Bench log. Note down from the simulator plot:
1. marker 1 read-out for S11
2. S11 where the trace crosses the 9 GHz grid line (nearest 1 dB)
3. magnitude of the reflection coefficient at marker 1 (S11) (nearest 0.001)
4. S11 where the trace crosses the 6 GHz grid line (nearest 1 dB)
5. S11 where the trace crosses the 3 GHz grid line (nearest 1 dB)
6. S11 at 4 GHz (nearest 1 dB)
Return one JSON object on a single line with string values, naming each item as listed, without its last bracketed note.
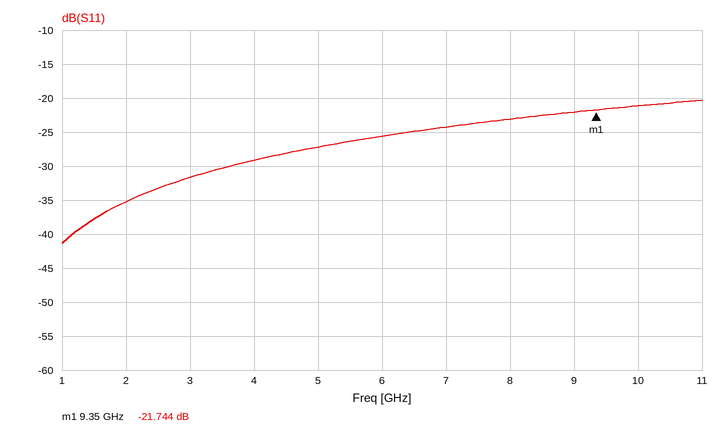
{"marker 1 read-out for S11": "-21.744 dB", "S11 where the trace crosses the 9 GHz grid line": "-22 dB", "magnitude of the reflection coefficient at marker 1 (S11)": "0.082", "S11 where the trace crosses the 6 GHz grid line": "-26 dB", "S11 where the trace crosses the 3 GHz grid line": "-32 dB", "S11 at 4 GHz": "-29 dB"}
